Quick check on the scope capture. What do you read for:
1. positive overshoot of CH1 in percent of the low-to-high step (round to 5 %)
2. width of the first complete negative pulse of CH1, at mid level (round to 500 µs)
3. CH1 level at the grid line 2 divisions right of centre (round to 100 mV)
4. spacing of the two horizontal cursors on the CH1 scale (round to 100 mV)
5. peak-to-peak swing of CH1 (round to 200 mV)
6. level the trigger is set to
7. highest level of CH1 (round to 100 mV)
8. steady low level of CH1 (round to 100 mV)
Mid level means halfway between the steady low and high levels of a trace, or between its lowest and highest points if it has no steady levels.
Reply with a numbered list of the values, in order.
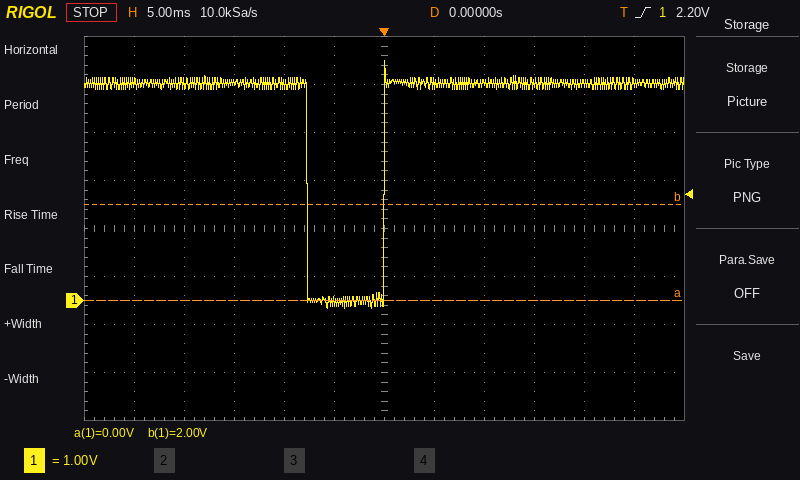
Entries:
1. 10 %
2. 7.5 ms
3. 4.5 V
4. 2.0 V
5. 5.2 V
6. 2.20 V
7. 5.0 V
8. 0.0 V
